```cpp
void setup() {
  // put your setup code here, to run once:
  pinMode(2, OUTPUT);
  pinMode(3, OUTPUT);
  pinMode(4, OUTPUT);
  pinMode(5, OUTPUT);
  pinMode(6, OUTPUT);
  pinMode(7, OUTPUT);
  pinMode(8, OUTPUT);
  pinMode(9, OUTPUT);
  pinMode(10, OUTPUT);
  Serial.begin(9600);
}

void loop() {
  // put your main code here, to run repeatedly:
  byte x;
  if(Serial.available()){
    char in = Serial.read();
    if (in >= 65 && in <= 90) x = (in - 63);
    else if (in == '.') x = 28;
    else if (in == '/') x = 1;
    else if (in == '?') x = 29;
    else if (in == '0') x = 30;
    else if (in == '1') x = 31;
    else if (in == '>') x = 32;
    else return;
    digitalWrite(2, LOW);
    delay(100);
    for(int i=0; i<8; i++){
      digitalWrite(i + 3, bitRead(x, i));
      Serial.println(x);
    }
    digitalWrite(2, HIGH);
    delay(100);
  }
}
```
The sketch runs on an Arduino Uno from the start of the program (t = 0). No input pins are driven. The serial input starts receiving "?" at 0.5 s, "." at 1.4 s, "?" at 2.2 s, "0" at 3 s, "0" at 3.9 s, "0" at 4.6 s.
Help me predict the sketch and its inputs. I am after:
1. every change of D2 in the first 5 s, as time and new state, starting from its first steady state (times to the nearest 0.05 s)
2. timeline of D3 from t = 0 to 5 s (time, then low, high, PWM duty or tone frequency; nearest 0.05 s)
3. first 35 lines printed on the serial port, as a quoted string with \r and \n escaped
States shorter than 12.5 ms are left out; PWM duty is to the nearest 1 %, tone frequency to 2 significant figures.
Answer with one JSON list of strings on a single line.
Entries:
["0 s low; 0.6 s high; 1.4 s low; 1.5 s high; 2.2 s low; 2.3 s high; 3 s low; 3.1 s high; 3.9 s low; 4 s high; 4.6 s low; 4.7 s high", "0 s low; 0.6 s high; 1.5 s low; 2.3 s high; 3.1 s low", "\"29\\r\\n29\\r\\n29\\r\\n29\\r\\n29\\r\\n29\\r\\n29\\r\\n29\\r\\n28\\r\\n28\\r\\n28\\r\\n28\\r\\n28\\r\\n28\\r\\n28\\r\\n28\\r\\n29\\r\\n29\\r\\n29\\r\\n29\\r\\n29\\r\\n29\\r\\n29\\r\\n29\\r\\n30\\r\\n30\\r\\n30\\r\\n30\\r\\n30\\r\\n30\\r\\n30\\r\\n30\\r\\n30\\r\\n30\\r\\n30\\r\\n\""]
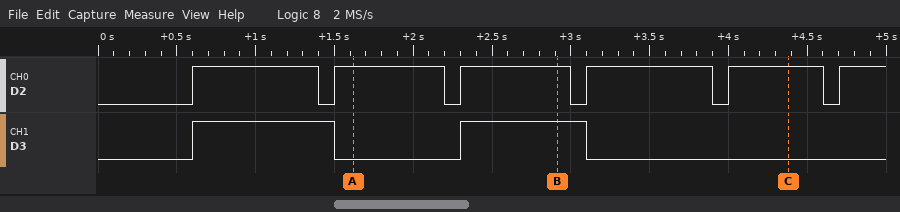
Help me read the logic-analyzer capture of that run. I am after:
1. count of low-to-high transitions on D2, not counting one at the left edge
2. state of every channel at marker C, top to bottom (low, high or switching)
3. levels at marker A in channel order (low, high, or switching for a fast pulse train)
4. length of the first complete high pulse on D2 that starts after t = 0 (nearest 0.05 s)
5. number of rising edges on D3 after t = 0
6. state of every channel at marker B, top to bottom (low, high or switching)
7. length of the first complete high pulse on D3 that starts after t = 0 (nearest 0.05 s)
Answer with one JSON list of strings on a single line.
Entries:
["6", "D2 high, D3 low", "D2 high, D3 low", "0.80 s", "2", "D2 high, D3 high", "0.90 s"]
